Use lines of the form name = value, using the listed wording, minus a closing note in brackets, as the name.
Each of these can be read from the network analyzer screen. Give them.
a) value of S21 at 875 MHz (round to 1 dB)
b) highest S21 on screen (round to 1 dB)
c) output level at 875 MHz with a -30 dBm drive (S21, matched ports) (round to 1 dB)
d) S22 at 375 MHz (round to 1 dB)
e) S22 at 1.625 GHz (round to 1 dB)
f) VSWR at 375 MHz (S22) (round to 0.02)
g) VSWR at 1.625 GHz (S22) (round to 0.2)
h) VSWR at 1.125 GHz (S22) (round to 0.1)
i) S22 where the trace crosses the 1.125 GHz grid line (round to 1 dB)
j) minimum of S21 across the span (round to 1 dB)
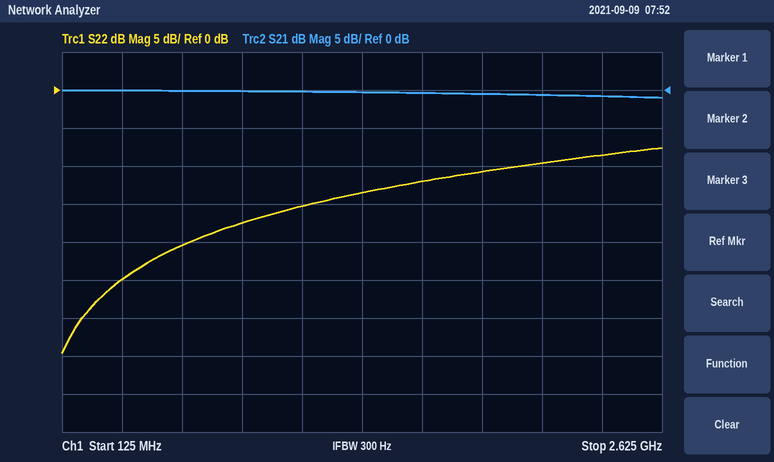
value of S21 at 875 MHz = 0 dB
highest S21 on screen = 0 dB
output level at 875 MHz with a -30 dBm drive (S21, matched ports) = -30 dBm
S22 at 375 MHz = -25 dB
S22 at 1.625 GHz = -12 dB
VSWR at 375 MHz (S22) = 1.12
VSWR at 1.625 GHz (S22) = 1.6
VSWR at 1.125 GHz (S22) = 1.4
S22 where the trace crosses the 1.125 GHz grid line = -15 dB
minimum of S21 across the span = -1 dB
